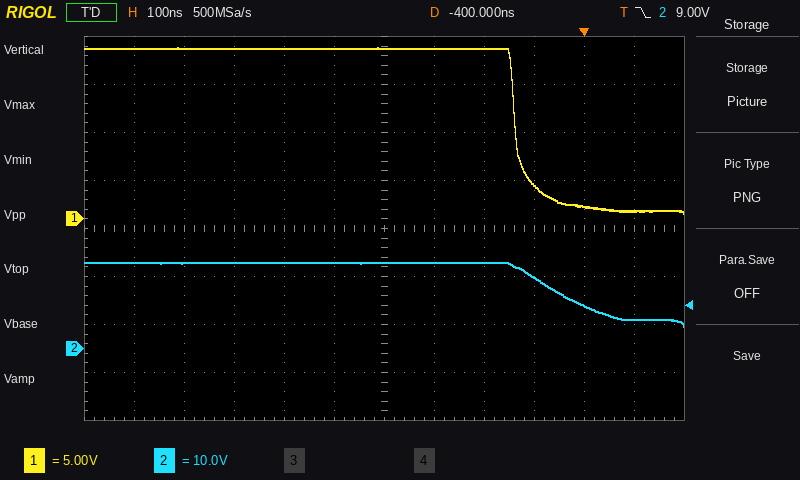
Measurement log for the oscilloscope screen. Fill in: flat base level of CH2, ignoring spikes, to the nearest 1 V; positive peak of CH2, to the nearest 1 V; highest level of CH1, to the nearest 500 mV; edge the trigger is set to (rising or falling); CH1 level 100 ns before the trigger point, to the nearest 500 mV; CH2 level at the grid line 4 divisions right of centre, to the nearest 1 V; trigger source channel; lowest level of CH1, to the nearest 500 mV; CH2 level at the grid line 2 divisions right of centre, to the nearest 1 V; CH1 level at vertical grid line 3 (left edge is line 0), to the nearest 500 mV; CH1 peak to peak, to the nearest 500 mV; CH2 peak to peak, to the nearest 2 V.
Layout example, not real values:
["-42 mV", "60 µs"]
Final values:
["6 V", "18 V", "18.0 V", "falling", "3.5 V", "9 V", "CH2", "500 mV", "18 V", "18.0 V", "17.5 V", "14 V"]
